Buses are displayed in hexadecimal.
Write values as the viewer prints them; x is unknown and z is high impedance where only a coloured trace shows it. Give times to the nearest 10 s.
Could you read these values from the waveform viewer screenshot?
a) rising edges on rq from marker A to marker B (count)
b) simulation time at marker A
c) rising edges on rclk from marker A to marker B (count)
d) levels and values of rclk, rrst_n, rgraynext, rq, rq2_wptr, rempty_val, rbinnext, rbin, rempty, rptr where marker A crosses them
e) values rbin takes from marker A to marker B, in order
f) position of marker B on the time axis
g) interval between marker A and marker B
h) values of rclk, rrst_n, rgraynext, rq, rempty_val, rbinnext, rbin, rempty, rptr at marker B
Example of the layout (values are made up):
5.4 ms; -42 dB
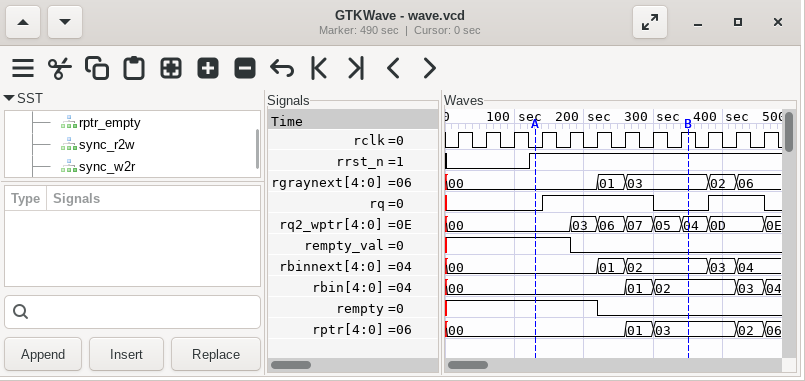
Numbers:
1; 130 s; 6; rclk=0, rrst_n=1, rgraynext=00, rq=0, rq2_wptr=00, rempty_val=1, rbinnext=00, rbin=00, rempty=1, rptr=00; 00, 01, 02; 350 s; 220 s; rclk=1, rrst_n=1, rgraynext=03, rq=0, rempty_val=0, rbinnext=02, rbin=02, rempty=0, rptr=03
